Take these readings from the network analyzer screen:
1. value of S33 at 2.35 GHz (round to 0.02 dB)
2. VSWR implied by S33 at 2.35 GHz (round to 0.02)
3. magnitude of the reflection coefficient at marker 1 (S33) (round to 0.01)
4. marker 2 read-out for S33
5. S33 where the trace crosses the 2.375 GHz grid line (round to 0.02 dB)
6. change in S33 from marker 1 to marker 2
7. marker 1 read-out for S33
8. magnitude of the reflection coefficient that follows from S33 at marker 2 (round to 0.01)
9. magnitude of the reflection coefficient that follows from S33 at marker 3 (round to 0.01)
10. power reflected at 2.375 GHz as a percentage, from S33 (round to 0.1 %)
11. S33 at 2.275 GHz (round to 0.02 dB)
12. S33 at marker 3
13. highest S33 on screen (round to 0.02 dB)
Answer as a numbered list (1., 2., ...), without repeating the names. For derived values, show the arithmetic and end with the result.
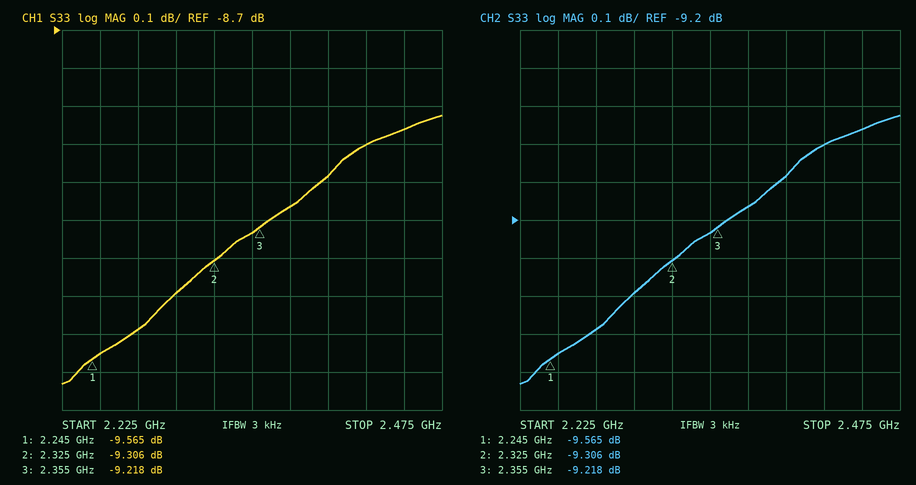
1. -9.24 dB
2. |Γ| = 10^(-9.24/20) = 0.3451; VSWR = (1 + 0.3451)/(1 − 0.3451) ≈ 2.05, so 2.06 to the nearest 0.02
3. 10^(-9.565/20) ≈ 0.33
4. -9.306 dB
5. -9.16 dB
6. -9.306 − (-9.565) = 0.259 dB
7. -9.565 dB
8. 10^(-9.306/20) ≈ 0.34
9. 10^(-9.218/20) ≈ 0.35
10. 10^(-9.16/10) ≈ 12.1 %
11. -9.48 dB
12. -9.218 dB
13. -8.92 dB
